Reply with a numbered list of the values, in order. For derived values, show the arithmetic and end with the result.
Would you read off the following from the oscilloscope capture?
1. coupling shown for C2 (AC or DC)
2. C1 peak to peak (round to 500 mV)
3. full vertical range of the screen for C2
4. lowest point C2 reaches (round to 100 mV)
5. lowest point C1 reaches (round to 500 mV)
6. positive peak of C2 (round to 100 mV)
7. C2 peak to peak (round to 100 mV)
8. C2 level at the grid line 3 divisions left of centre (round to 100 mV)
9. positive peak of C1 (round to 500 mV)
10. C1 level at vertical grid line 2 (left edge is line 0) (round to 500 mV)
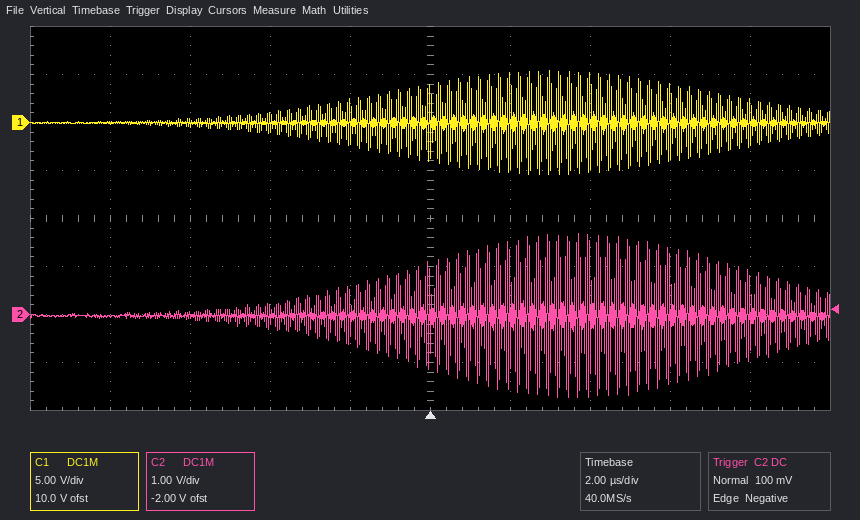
1. DC
2. 5.5 V − (-5.5 V) = 11.0 V
3. 8 V
4. -1.7 V
5. -5.5 V
6. 1.7 V
7. 1.7 V − (-1.7 V) = 3.4 V
8. 0.0 V
9. 5.5 V
10. 0.0 V
